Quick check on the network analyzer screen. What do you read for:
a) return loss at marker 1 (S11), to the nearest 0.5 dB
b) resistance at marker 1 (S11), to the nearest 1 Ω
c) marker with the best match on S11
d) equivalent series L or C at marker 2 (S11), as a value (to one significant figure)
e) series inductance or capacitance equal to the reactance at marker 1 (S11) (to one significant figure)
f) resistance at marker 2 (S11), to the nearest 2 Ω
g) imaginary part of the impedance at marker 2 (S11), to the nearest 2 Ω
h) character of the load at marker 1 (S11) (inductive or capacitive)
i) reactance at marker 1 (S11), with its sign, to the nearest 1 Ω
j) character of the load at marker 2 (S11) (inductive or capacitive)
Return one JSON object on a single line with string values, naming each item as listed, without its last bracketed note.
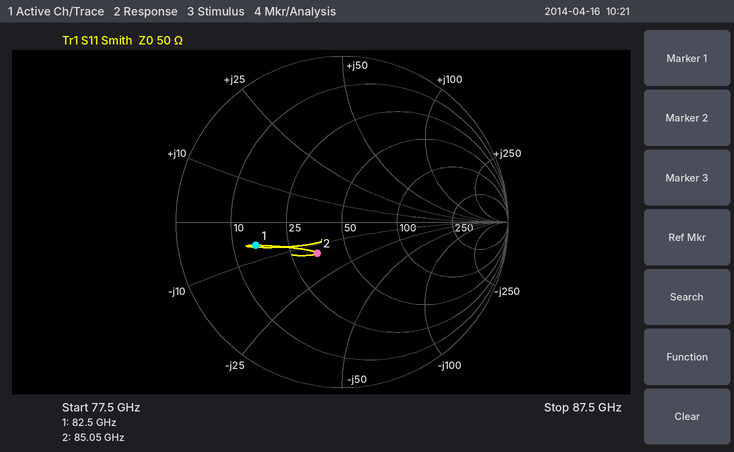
{"return loss at marker 1 (S11), to the nearest 0.5 dB": "5.5 dB", "resistance at marker 1 (S11), to the nearest 1 Ω": "15 Ω", "marker with the best match on S11": "marker 2", "equivalent series L or C at marker 2 (S11), as a value": "100 fF", "series inductance or capacitance equal to the reactance at marker 1 (S11)": "300 fF", "resistance at marker 2 (S11), to the nearest 2 Ω": "34 Ω", "imaginary part of the impedance at marker 2 (S11), to the nearest 2 Ω": "-14 Ω", "character of the load at marker 1 (S11)": "capacitive", "reactance at marker 1 (S11), with its sign, to the nearest 1 Ω": "-6 Ω", "character of the load at marker 2 (S11)": "capacitive"}
